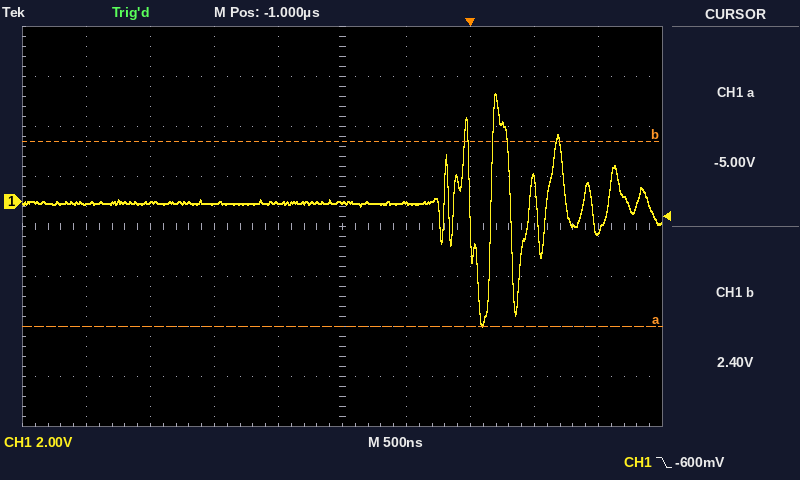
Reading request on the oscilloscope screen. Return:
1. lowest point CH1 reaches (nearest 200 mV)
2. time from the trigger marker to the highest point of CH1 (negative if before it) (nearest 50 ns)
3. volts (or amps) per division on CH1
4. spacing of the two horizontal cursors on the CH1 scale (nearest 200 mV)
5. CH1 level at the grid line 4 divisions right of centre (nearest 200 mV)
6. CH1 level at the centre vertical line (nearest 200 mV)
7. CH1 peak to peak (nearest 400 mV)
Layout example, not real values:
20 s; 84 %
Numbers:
-5.0 V; +200 ns; 2 V; 7.4 V; -1.2 V; 0.0 V; 9.2 V
